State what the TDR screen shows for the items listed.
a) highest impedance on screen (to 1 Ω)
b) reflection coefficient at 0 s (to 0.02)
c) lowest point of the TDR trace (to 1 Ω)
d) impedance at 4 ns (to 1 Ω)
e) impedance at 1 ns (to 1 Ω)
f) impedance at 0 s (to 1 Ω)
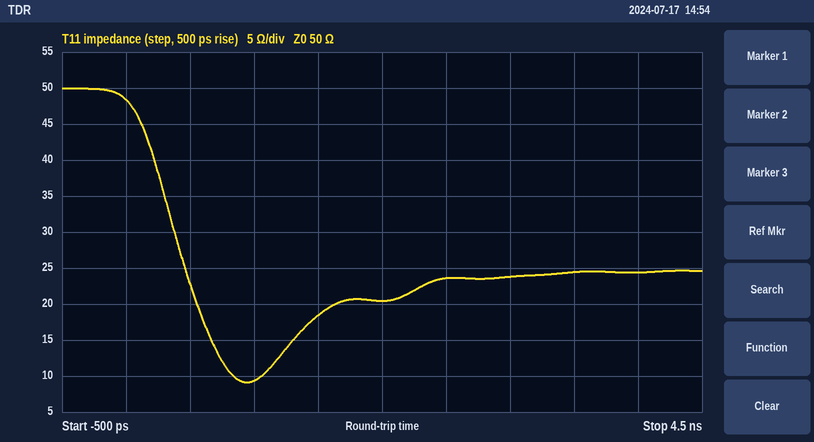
50 Ω
-0.02
9 Ω
24 Ω
9 Ω
48 Ω
